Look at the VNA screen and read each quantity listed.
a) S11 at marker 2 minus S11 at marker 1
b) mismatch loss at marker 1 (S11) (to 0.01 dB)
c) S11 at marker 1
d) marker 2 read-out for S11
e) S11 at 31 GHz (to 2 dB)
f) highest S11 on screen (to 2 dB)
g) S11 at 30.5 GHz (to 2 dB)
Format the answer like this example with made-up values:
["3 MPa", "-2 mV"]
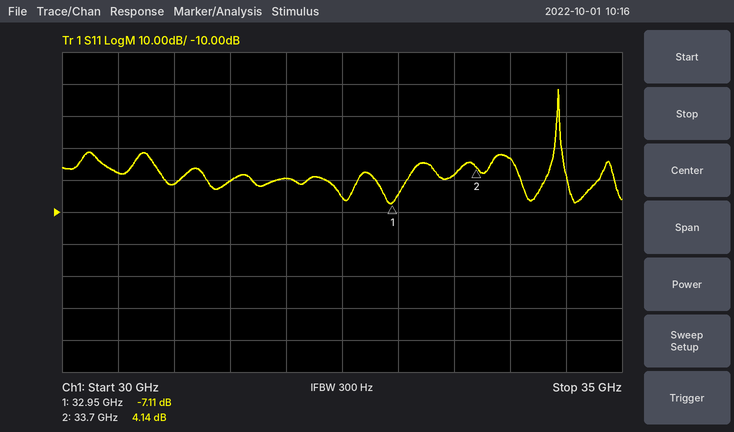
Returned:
["11.25 dB", "0.94 dB", "-7.11 dB", "4.14 dB", "-2 dB", "28 dB", "2 dB"]
